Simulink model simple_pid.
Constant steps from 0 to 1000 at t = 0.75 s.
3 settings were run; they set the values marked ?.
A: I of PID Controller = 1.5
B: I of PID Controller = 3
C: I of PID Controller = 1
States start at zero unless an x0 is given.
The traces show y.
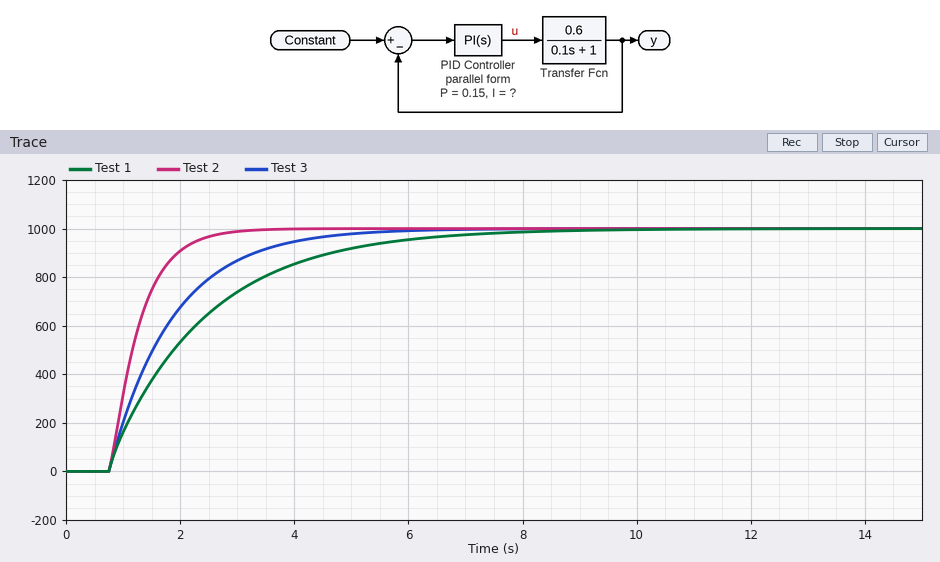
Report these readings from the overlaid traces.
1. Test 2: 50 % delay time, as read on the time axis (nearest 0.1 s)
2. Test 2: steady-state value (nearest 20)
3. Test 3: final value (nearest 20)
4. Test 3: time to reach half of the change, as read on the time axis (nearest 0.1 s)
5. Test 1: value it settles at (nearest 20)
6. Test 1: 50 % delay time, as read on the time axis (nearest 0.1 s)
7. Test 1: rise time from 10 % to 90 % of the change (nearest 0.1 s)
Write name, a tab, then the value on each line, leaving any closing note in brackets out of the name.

Test 2: 50 % delay time, as read on the time axis	1.2 s
Test 2: steady-state value	1000
Test 3: final value	1000
Test 3: time to reach half of the change, as read on the time axis	1.5 s
Test 1: value it settles at	1000
Test 1: 50 % delay time, as read on the time axis	1.9 s
Test 1: rise time from 10 % to 90 % of the change	3.8 s
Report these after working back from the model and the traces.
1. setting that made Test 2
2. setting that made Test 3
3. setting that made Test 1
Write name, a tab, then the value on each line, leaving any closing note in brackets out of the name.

setting that made Test 2	B
setting that made Test 3	A
setting that made Test 1	C
